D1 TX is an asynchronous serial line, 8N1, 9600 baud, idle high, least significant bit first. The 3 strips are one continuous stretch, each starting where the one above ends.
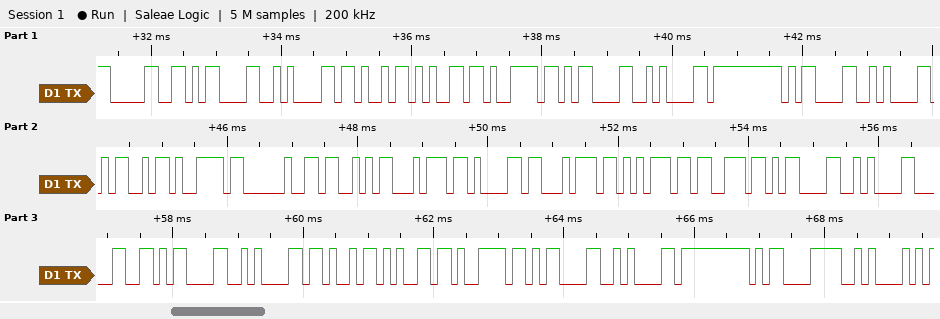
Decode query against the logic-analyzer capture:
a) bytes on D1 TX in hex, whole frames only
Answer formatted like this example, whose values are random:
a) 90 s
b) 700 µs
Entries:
a) 30 0D 0A 4B 65 79 0D 0A FF 0D 0A 4D 79 20 53 74 61 74 75 73 0D 0A 30 0D 0A 4B 65 79 0D 0A FF 0D 0A
